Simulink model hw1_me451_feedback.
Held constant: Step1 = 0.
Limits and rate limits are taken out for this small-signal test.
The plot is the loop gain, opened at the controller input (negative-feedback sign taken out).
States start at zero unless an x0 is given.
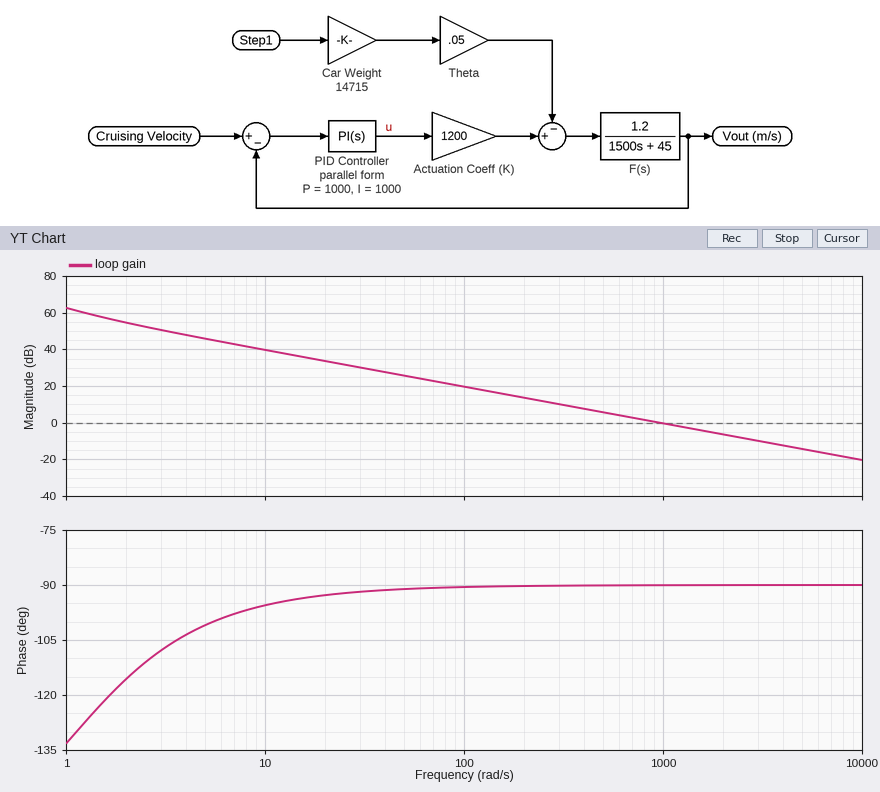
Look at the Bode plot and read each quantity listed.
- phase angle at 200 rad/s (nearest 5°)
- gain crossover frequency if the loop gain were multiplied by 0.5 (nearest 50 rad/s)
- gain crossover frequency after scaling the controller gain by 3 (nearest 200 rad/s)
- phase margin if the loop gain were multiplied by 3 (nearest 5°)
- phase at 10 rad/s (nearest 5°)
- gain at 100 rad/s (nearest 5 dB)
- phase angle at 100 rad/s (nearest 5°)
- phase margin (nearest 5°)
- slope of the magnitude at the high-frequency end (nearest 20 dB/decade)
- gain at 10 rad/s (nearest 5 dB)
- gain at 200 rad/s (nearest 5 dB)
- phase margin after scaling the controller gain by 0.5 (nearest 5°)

-90°
500 rad/s
2800 rad/s
90°
-95°
20 dB
-90°
90°
-20 dB/decade
40 dB
15 dB
90°
